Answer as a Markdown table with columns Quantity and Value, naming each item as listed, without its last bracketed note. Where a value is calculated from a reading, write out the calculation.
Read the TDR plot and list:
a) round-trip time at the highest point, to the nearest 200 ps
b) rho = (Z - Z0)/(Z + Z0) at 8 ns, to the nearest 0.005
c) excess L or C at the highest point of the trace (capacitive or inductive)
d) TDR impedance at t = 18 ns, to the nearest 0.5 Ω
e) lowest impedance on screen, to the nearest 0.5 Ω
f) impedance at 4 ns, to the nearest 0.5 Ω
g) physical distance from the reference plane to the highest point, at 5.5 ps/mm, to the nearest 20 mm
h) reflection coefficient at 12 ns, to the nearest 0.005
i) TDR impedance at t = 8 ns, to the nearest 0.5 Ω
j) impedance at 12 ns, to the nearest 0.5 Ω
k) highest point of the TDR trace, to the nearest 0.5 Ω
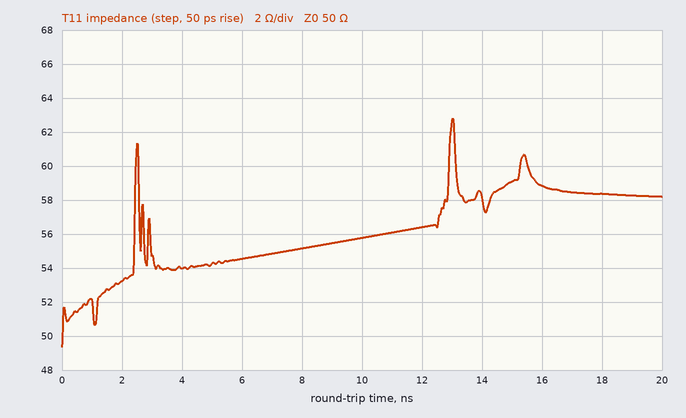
| Quantity | Value |
|---|---|
| round-trip time at the highest point, to the nearest 200 ps | 13.0 ns |
| rho = (Z - Z0)/(Z + Z0) at 8 ns, to the nearest 0.005 | (55 − 50)/(55 + 50) ≈ +0.0476, so +0.050 to the nearest 0.005 |
| excess L or C at the highest point of the trace | inductive |
| TDR impedance at t = 18 ns, to the nearest 0.5 Ω | 58.5 Ω |
| lowest impedance on screen, to the nearest 0.5 Ω | 49.5 Ω |
| impedance at 4 ns, to the nearest 0.5 Ω | 54.0 Ω |
| physical distance from the reference plane to the highest point, at 5.5 ps/mm, to the nearest 20 mm | 13.0 ns / 2 / 5.5 ps/mm ≈ 1.18 m |
| reflection coefficient at 12 ns, to the nearest 0.005 | (56.5 − 50)/(56.5 + 50) ≈ +0.0610, so +0.060 to the nearest 0.005 |
| TDR impedance at t = 8 ns, to the nearest 0.5 Ω | 55.0 Ω |
| impedance at 12 ns, to the nearest 0.5 Ω | 56.5 Ω |
| highest point of the TDR trace, to the nearest 0.5 Ω | 63.0 Ω |
